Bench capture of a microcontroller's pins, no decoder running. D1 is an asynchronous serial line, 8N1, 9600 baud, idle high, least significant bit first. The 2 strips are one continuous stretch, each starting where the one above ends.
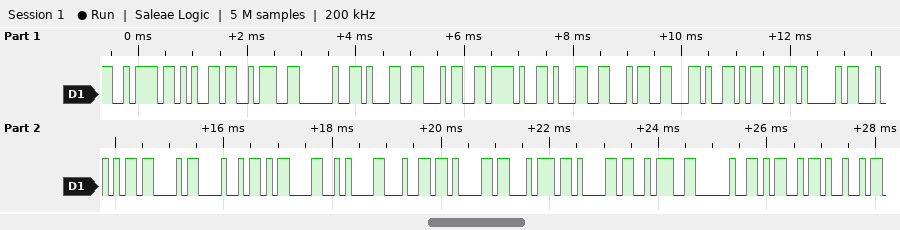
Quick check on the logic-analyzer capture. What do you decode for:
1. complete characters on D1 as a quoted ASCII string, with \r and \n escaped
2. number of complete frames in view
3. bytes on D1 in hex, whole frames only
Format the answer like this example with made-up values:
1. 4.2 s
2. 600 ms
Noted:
1. "ze: 14/14,MATCH\r\ndata: MI"
2. 25
3. 7A 65 3A 20 31 34 2F 31 34 2C 4D 41 54 43 48 0D 0A 64 61 74 61 3A 20 4D 49
